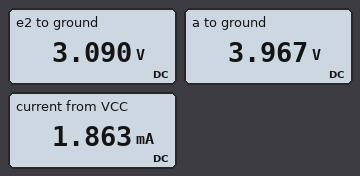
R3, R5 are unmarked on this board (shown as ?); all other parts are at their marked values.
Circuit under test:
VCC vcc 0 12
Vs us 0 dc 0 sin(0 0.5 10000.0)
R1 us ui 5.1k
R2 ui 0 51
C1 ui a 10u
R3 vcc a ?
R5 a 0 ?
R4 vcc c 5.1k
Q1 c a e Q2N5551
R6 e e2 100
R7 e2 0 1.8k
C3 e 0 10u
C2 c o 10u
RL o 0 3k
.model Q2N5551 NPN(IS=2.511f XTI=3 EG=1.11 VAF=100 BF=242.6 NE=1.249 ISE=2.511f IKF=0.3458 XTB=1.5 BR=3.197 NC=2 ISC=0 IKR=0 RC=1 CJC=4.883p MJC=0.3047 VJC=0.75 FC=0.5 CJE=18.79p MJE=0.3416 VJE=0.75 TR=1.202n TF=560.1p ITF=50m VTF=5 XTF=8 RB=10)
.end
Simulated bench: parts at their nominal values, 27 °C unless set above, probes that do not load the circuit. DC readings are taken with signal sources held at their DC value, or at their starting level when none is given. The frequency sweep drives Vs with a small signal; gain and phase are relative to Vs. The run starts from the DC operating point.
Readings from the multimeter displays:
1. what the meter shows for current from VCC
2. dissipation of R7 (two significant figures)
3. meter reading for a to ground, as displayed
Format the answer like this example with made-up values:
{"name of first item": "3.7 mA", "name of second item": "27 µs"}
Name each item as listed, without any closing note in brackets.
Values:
{"what the meter shows for current from VCC": "1.863 mA", "dissipation of R7": "5.3 mW", "meter reading for a to ground, as displayed": "3.967 V"}
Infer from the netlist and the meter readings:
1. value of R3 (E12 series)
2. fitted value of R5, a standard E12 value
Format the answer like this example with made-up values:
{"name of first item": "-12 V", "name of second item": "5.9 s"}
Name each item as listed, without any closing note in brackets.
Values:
{"value of R3": "47 kΩ", "fitted value of R5, a standard E12 value": "27 kΩ"}
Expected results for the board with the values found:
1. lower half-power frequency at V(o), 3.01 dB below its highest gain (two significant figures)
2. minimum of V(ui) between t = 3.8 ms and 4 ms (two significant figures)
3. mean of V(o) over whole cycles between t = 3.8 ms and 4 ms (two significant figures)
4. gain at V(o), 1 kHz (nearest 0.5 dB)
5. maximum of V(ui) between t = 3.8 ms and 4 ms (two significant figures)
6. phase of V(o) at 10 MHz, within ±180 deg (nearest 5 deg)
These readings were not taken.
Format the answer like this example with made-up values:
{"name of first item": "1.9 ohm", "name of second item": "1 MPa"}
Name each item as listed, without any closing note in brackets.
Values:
{"lower half-power frequency at V(o), 3.01 dB below its highest gain": "390 Hz", "minimum of V(ui) between t = 3.8 ms and 4 ms": "-4.4 mV", "mean of V(o) over whole cycles between t = 3.8 ms and 4 ms": "48 mV", "gain at V(o), 1 kHz": "-15.5 dB", "maximum of V(ui) between t = 3.8 ms and 4 ms": "2.6 mV", "phase of V(o) at 10 MHz, within ±180 deg": "135 deg"}
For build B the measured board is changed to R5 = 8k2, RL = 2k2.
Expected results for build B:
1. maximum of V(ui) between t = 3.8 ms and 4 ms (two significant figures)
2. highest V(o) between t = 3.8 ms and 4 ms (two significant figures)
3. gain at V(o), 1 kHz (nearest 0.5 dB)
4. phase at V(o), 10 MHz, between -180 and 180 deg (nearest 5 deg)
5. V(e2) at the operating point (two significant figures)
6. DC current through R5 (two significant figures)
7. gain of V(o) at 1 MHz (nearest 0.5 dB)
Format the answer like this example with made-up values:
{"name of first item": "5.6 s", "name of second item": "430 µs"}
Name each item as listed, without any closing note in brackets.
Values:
{"maximum of V(ui) between t = 3.8 ms and 4 ms": "4.9 mV", "highest V(o) between t = 3.8 ms and 4 ms": "150 mV", "gain at V(o), 1 kHz": "-10.5 dB", "phase at V(o), 10 MHz, between -180 and 180 deg": "145 deg", "V(e2) at the operating point": "1.0 V", "DC current through R5": "210 µA", "gain of V(o) at 1 MHz": "-10.0 dB"}
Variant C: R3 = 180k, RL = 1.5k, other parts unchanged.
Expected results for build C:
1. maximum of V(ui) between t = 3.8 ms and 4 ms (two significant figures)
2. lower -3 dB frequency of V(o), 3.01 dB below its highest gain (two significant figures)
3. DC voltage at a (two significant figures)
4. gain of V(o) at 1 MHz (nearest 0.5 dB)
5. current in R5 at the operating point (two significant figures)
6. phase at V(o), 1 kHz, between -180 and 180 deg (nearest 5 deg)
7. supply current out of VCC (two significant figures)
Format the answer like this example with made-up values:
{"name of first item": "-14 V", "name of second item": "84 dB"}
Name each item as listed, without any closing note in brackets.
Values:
{"maximum of V(ui) between t = 3.8 ms and 4 ms": "4.9 mV", "lower -3 dB frequency of V(o), 3.01 dB below its highest gain": "270 Hz", "DC voltage at a": "1.5 V", "gain of V(o) at 1 MHz": "-14.5 dB", "current in R5 at the operating point": "55 µA", "phase at V(o), 1 kHz, between -180 and 180 deg": "-165 deg", "supply current out of VCC": "480 µA"}
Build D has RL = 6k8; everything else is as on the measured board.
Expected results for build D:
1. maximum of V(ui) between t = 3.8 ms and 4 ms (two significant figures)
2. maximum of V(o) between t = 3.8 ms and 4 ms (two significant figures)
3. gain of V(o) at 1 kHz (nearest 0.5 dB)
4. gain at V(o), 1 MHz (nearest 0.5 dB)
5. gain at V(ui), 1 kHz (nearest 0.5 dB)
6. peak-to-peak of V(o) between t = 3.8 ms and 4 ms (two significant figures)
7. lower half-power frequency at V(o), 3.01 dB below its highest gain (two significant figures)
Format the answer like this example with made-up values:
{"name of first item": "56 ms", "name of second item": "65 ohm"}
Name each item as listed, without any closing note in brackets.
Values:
{"maximum of V(ui) between t = 3.8 ms and 4 ms": "2.5 mV", "maximum of V(o) between t = 3.8 ms and 4 ms": "450 mV", "gain of V(o) at 1 kHz": "-15.0 dB", "gain at V(o), 1 MHz": "-14.5 dB", "gain at V(ui), 1 kHz": "-43.5 dB", "peak-to-peak of V(o) between t = 3.8 ms and 4 ms": "510 mV", "lower half-power frequency at V(o), 3.01 dB below its highest gain": "350 Hz"}
